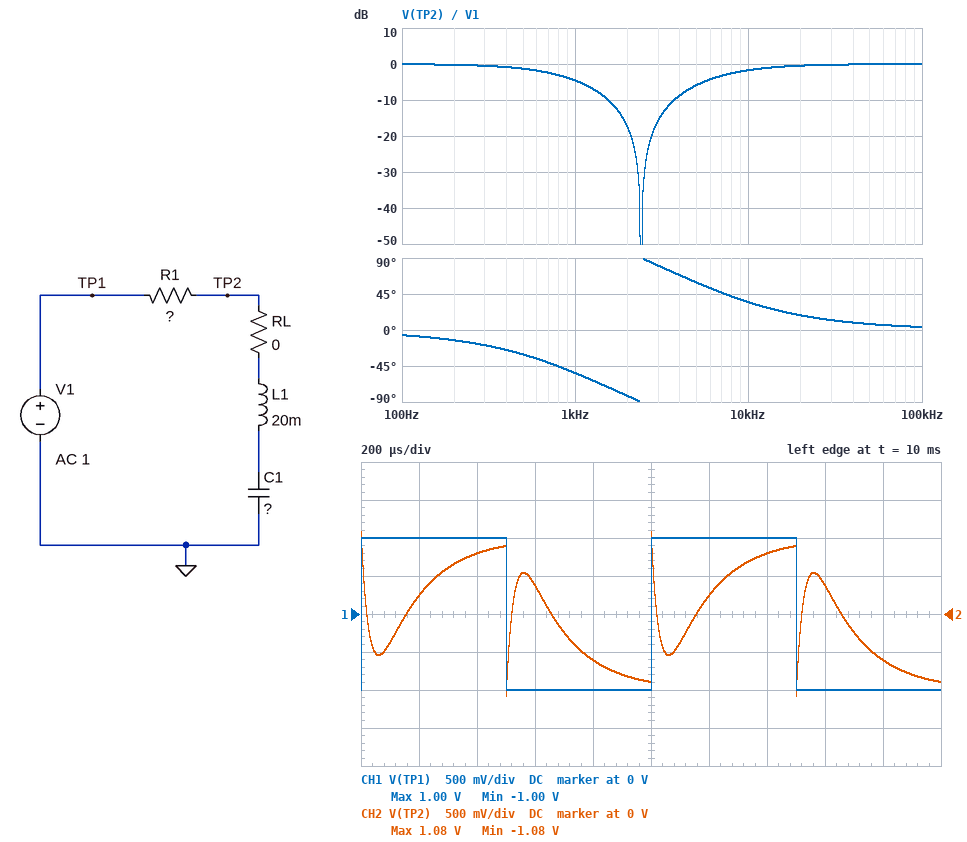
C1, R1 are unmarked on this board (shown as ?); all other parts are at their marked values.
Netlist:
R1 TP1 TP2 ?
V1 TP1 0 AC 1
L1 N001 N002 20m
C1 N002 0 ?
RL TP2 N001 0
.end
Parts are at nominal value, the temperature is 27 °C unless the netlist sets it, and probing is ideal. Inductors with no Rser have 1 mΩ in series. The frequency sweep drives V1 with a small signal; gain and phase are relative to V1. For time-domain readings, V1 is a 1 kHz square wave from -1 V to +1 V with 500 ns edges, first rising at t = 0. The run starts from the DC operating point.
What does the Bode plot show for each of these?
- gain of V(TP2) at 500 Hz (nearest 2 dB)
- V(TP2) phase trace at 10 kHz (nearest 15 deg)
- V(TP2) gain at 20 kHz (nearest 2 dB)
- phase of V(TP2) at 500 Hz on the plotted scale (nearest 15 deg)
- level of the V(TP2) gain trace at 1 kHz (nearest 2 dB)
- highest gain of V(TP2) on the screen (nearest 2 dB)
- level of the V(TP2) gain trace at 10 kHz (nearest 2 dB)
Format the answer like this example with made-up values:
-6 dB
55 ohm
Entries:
-2 dB
30 deg
0 dB
-30 deg
-4 dB
0 dB
-2 dB
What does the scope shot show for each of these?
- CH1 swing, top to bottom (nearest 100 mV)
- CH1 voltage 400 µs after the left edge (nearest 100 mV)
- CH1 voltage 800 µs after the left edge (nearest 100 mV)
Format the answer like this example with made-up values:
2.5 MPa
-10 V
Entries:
2.0 V
1.0 V
-1.0 V
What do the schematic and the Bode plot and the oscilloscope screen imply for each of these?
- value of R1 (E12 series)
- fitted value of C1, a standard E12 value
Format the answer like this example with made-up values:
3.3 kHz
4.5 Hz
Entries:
820 Ω
220 nF
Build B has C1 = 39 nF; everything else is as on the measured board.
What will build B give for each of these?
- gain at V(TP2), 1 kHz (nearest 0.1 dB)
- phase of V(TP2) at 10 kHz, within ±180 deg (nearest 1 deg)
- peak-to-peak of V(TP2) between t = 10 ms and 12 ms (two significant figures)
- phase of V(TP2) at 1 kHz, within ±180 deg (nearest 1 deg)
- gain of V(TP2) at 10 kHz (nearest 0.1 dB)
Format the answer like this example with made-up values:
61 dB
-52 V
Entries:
-0.2 dB
44 deg
2.3 V
-12 deg
-2.9 dB
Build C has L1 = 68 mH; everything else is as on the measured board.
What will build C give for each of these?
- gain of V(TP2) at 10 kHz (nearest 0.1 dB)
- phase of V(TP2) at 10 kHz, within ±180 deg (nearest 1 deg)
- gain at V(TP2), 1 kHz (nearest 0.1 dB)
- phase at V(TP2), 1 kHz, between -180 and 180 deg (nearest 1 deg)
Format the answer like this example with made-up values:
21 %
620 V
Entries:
-0.2 dB
11 deg
-9.4 dB
-70 deg
